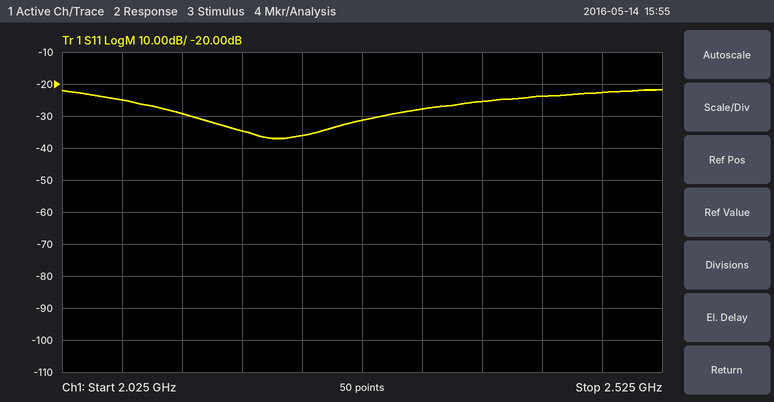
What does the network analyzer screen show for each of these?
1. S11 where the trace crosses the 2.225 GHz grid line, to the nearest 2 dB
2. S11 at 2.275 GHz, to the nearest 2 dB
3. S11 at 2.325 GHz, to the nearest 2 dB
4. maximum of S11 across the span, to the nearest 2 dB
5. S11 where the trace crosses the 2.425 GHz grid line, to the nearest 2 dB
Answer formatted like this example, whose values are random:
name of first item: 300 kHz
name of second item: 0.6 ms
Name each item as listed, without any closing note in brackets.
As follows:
S11 where the trace crosses the 2.225 GHz grid line, to the nearest 2 dB: -36 dB
S11 at 2.275 GHz, to the nearest 2 dB: -32 dB
S11 at 2.325 GHz, to the nearest 2 dB: -28 dB
maximum of S11 across the span, to the nearest 2 dB: -22 dB
S11 where the trace crosses the 2.425 GHz grid line, to the nearest 2 dB: -24 dB
